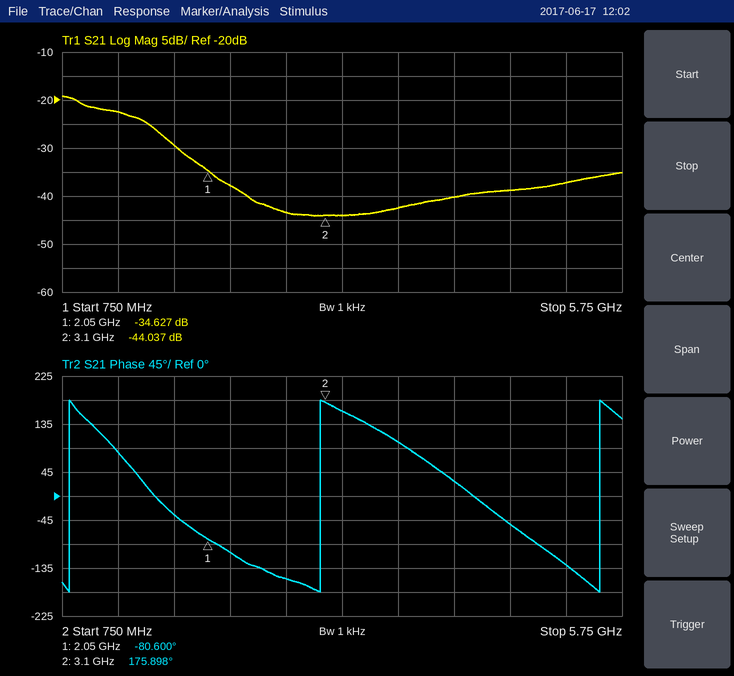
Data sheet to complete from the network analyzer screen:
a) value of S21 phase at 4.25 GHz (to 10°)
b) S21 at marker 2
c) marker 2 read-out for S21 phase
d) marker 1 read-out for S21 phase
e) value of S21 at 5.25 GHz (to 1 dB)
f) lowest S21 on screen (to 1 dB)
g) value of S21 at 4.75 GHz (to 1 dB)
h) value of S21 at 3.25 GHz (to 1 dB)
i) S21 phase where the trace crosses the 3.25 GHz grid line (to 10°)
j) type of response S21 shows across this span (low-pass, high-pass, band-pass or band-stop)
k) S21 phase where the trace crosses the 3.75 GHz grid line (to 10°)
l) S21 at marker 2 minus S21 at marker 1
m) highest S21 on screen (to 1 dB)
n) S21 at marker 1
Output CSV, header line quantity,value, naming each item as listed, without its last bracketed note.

quantity,value
value of S21 phase at 4.25 GHz,30°
S21 at marker 2,-44.037 dB
marker 2 read-out for S21 phase,175.898°
marker 1 read-out for S21 phase,-80.600°
value of S21 at 5.25 GHz,-37 dB
lowest S21 on screen,-44 dB
value of S21 at 4.75 GHz,-39 dB
value of S21 at 3.25 GHz,-44 dB
S21 phase where the trace crosses the 3.25 GHz grid line,160°
type of response S21 shows across this span,low-pass
S21 phase where the trace crosses the 3.75 GHz grid line,100°
S21 at marker 2 minus S21 at marker 1,-9.410 dB
highest S21 on screen,-19 dB
S21 at marker 1,-34.627 dB
